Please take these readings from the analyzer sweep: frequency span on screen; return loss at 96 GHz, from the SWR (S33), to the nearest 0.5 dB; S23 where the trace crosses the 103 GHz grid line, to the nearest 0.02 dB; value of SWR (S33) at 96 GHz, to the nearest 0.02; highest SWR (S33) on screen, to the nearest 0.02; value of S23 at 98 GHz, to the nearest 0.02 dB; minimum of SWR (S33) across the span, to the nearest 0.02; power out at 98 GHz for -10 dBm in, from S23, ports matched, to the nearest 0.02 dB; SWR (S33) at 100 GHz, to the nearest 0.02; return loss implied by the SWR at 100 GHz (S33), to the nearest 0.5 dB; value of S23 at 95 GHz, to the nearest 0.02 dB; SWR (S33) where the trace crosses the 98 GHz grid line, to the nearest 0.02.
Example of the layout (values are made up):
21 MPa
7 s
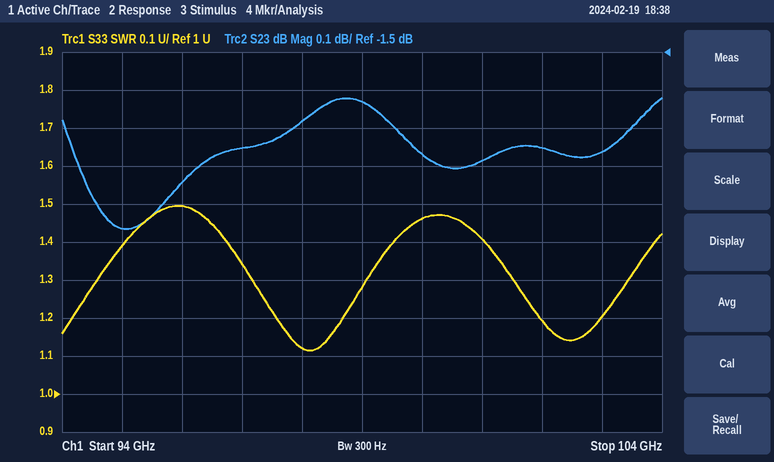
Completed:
10 GHz
14.0 dB
-1.76 dB
1.50
1.50
-1.68 dB
1.12
-11.68 dBm
1.46
14.5 dB
-1.96 dB
1.12
